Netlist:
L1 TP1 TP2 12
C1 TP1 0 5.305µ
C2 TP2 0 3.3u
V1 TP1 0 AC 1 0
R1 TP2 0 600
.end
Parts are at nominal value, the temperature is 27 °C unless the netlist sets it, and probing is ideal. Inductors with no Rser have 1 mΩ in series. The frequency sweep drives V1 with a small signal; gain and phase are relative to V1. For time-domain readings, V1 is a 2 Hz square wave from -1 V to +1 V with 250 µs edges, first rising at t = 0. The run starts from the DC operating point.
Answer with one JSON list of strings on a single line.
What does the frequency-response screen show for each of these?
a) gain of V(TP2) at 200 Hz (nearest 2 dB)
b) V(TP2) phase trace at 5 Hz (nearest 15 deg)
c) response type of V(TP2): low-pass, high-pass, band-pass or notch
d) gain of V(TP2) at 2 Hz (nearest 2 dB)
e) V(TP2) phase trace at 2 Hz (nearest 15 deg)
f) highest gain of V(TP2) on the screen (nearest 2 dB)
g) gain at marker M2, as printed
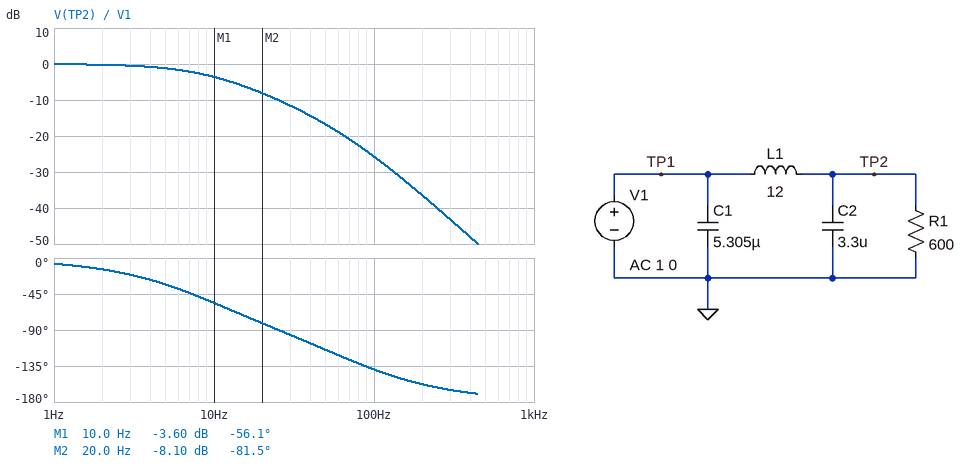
["-36 dB", "-30 deg", "low-pass", "0 dB", "-15 deg", "0 dB", "-8.10 dB"]
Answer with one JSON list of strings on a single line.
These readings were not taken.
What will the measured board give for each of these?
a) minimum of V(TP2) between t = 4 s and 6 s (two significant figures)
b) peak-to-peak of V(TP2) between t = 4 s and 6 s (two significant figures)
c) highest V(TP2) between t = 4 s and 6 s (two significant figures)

["-1.0 V", "2.0 V", "1.0 V"]
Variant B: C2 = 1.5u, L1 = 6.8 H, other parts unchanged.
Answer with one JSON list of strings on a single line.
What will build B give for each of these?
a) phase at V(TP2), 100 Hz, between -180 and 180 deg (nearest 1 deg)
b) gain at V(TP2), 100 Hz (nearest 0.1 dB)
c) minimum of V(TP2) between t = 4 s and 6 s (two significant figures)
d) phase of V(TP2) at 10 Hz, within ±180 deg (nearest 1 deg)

["-113 deg", "-17.8 dB", "-1.0 V", "-37 deg"]
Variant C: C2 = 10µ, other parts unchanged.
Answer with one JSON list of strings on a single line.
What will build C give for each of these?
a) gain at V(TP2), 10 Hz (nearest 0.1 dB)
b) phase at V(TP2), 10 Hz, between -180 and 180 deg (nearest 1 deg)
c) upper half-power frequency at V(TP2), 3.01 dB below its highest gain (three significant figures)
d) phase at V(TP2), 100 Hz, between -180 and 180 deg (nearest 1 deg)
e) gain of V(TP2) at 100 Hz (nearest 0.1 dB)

["-2.7 dB", "-67 deg", "10.6 Hz", "-165 deg", "-33.6 dB"]
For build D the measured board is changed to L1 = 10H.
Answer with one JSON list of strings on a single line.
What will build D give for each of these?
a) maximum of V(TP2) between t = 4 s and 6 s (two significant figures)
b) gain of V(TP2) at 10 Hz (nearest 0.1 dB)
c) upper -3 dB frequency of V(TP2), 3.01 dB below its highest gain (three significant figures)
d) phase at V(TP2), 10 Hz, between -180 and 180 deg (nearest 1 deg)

["1.0 V", "-2.7 dB", "10.8 Hz", "-50 deg"]
